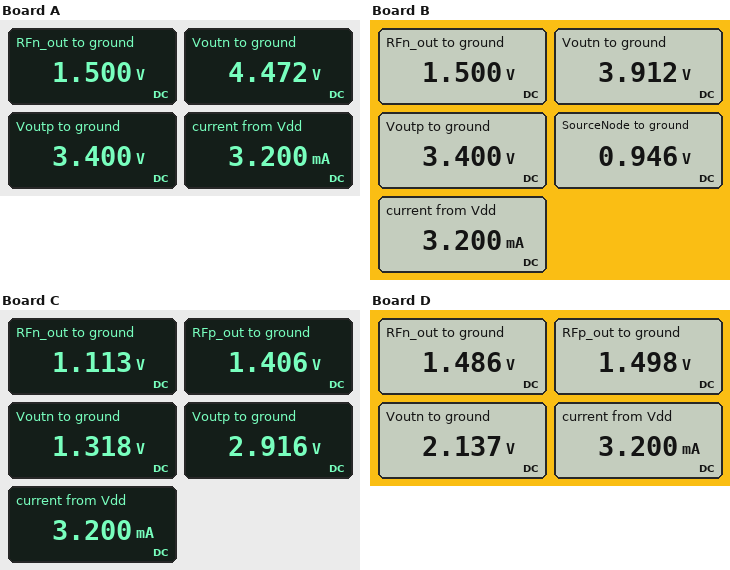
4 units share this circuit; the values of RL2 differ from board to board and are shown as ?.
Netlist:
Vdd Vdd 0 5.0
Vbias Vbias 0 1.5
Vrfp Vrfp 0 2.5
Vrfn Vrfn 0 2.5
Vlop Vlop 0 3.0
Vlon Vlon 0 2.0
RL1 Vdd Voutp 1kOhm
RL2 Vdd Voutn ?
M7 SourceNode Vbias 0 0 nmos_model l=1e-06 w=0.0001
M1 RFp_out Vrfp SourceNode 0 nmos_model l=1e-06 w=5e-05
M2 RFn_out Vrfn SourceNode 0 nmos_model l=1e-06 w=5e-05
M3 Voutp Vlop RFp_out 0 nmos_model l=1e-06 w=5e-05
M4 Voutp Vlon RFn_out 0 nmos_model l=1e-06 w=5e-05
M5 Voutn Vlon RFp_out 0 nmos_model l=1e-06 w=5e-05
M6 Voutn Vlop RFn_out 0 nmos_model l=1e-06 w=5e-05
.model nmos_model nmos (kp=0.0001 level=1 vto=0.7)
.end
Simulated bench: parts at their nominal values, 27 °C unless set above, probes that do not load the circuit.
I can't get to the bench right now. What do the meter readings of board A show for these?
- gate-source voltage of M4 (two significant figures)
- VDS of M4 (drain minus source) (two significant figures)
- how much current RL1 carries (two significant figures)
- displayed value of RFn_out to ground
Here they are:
500 mV
1.9 V
1.6 mA
1.500 V
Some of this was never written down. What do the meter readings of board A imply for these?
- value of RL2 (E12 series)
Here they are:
330 Ω
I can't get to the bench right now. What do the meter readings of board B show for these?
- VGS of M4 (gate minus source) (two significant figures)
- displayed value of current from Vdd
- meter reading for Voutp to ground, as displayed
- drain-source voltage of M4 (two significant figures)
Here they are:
500 mV
3.200 mA
3.400 V
1.9 V
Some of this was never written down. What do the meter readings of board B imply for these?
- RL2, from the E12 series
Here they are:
680 Ω
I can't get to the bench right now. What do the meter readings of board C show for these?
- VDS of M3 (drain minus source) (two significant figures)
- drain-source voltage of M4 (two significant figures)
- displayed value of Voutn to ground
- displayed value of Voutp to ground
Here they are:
1.5 V
1.8 V
1.318 V
2.916 V
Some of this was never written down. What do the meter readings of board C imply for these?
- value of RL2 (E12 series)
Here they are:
3.3 kΩ
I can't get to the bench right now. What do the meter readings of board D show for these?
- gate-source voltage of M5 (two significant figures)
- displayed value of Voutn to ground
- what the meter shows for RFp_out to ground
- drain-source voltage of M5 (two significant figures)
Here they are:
500 mV
2.137 V
1.498 V
640 mV
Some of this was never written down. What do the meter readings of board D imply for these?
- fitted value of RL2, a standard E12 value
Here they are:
1.8 kΩ
